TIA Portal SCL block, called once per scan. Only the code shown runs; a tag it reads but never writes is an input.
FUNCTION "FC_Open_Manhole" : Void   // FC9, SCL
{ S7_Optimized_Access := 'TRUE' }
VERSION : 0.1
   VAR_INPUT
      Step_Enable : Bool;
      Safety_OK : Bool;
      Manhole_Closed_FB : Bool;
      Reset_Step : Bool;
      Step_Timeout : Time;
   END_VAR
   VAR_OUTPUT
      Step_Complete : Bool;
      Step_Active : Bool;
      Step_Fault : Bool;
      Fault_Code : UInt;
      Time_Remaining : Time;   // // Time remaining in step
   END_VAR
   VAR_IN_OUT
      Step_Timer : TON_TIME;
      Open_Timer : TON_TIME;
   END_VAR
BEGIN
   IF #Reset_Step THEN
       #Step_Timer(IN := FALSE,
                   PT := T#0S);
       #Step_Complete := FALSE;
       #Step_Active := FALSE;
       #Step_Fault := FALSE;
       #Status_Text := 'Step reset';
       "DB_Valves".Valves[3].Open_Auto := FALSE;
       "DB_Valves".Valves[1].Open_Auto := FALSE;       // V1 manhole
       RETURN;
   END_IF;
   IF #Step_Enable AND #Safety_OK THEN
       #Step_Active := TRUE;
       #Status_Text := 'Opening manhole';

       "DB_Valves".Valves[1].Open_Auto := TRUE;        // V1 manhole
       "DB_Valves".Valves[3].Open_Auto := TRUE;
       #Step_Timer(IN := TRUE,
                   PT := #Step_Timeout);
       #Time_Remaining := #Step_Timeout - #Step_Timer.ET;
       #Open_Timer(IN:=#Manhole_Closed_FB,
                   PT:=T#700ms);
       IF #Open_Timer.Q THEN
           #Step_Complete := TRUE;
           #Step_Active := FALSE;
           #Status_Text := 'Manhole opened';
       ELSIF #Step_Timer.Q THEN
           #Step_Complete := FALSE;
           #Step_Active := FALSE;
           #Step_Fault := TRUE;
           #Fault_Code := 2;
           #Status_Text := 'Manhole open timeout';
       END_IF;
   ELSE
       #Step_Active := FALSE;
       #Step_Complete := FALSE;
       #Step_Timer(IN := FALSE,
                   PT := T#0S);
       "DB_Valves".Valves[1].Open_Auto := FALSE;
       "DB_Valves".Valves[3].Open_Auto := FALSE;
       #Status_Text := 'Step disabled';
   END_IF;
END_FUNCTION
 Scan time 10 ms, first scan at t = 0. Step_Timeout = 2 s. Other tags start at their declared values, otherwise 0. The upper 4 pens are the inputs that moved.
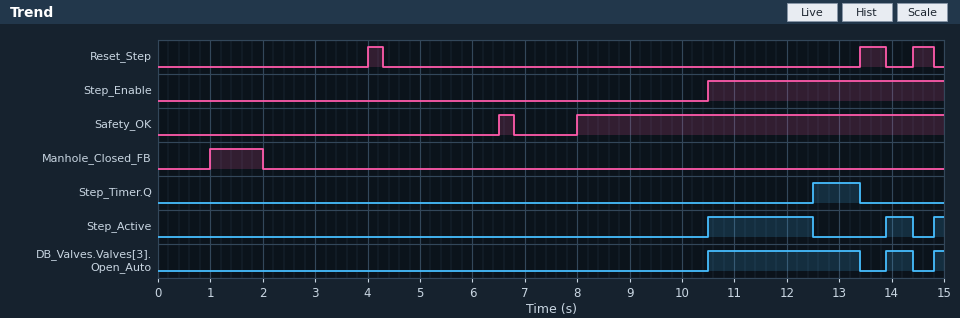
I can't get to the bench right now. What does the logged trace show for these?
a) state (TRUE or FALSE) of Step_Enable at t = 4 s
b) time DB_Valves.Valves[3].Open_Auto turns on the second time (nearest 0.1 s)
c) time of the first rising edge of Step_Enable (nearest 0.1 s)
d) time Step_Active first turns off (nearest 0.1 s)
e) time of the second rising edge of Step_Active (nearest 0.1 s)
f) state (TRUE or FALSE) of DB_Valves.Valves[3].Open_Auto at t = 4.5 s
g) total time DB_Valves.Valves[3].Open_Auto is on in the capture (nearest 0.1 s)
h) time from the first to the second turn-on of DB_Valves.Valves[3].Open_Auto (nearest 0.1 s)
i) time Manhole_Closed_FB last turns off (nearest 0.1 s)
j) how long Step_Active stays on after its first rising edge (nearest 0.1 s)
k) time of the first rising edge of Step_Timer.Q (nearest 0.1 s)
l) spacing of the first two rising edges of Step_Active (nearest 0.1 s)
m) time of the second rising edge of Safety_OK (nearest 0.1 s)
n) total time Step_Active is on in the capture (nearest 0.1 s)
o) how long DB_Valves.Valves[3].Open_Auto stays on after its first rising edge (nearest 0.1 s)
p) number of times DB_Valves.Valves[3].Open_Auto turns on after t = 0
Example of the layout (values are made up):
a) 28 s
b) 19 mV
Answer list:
a) FALSE
b) 13.9 s
c) 10.5 s
d) 12.5 s
e) 13.9 s
f) FALSE
g) 3.6 s
h) 3.4 s
i) 2.0 s
j) 2.0 s
k) 12.5 s
l) 3.4 s
m) 8.0 s
n) 2.7 s
o) 2.9 s
p) 3
